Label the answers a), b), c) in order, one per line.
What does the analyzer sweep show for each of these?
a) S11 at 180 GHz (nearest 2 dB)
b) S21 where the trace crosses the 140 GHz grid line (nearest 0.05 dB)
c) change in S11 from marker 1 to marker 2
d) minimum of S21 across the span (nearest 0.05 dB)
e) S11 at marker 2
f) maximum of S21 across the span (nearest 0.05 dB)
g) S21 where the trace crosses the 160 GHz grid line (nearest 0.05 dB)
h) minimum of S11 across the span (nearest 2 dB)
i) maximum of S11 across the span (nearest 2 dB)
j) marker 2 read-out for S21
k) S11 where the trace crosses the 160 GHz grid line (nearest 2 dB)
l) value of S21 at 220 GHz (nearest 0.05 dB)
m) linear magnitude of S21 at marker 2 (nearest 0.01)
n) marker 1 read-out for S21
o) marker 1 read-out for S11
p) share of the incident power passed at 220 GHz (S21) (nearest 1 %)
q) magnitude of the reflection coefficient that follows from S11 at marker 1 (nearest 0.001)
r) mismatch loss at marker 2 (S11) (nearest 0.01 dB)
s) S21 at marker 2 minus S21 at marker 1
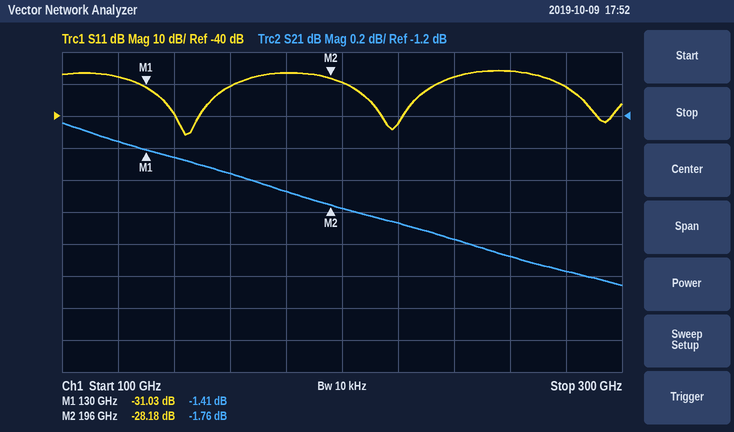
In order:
a) -26 dB
b) -1.45 dB
c) 2.85 dB
d) -2.25 dB
e) -28.18 dB
f) -1.25 dB
g) -1.55 dB
h) -46 dB
i) -26 dB
j) -1.76 dB
k) -30 dB
l) -1.85 dB
m) 0.82
n) -1.41 dB
o) -31.03 dB
p) 65 %
q) 0.028
r) 0.01 dB
s) -0.35 dB
